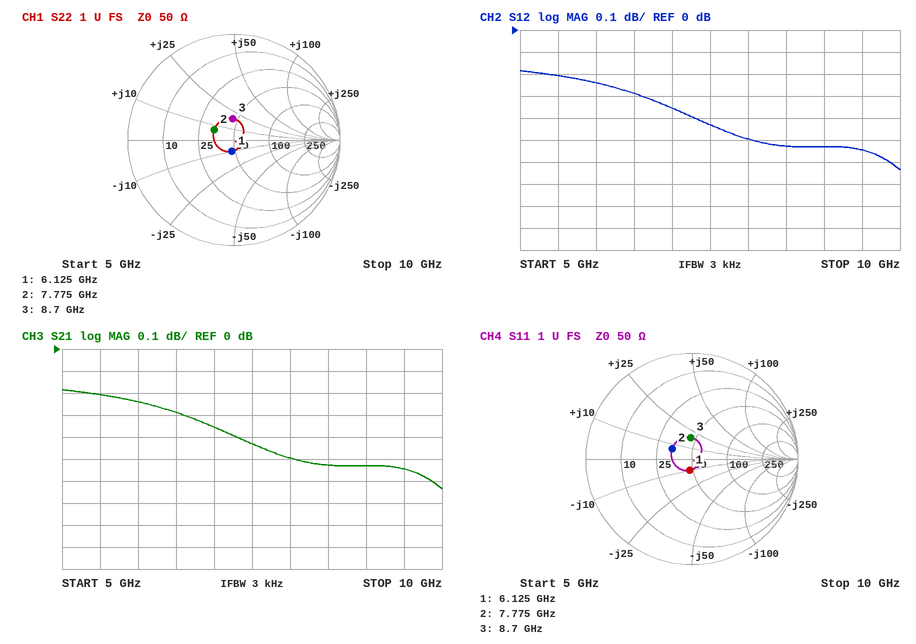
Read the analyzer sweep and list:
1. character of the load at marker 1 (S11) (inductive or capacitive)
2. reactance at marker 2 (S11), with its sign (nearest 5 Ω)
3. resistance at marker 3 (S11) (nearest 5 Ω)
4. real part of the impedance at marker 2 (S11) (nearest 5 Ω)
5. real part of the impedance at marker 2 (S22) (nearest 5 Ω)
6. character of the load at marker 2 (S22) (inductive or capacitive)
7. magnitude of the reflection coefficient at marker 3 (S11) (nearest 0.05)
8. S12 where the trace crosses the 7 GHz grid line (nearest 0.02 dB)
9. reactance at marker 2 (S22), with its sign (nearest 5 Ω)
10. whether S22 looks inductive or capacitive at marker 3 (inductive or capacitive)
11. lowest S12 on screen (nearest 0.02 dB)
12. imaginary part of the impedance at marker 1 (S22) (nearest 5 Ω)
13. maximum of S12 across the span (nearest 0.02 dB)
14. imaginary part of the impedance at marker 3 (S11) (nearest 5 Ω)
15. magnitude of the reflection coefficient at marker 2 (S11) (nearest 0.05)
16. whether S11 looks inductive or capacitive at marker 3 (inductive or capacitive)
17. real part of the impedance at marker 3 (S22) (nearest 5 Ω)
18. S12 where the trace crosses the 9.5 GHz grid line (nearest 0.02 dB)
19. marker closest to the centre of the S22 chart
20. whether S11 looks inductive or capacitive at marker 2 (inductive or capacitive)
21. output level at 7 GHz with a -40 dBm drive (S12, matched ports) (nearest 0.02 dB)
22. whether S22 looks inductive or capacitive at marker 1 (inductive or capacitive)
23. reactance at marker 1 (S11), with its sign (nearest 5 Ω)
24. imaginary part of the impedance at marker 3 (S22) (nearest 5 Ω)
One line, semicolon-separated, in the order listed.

capacitive; +5 Ω; 45 Ω; 35 Ω; 35 Ω; inductive; 0.20; -0.36 dB; +5 Ω; inductive; -0.64 dB; -10 Ω; -0.18 dB; +20 Ω; 0.20; inductive; 45 Ω; -0.54 dB; marker 1; inductive; -40.36 dBm; capacitive; -10 Ω; +20 Ω
